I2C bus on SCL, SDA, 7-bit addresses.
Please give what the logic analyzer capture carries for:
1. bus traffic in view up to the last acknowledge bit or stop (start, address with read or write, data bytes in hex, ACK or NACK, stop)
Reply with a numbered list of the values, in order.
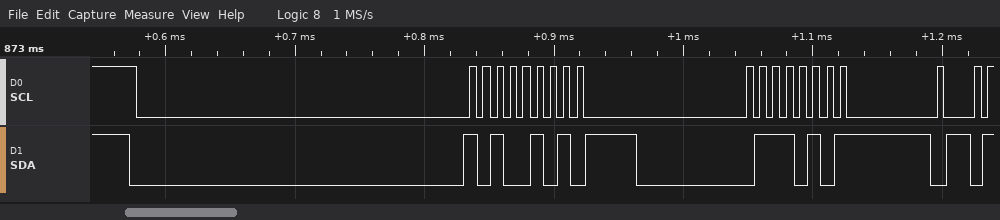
1. start, address 52 read ACK, 75 ACK
